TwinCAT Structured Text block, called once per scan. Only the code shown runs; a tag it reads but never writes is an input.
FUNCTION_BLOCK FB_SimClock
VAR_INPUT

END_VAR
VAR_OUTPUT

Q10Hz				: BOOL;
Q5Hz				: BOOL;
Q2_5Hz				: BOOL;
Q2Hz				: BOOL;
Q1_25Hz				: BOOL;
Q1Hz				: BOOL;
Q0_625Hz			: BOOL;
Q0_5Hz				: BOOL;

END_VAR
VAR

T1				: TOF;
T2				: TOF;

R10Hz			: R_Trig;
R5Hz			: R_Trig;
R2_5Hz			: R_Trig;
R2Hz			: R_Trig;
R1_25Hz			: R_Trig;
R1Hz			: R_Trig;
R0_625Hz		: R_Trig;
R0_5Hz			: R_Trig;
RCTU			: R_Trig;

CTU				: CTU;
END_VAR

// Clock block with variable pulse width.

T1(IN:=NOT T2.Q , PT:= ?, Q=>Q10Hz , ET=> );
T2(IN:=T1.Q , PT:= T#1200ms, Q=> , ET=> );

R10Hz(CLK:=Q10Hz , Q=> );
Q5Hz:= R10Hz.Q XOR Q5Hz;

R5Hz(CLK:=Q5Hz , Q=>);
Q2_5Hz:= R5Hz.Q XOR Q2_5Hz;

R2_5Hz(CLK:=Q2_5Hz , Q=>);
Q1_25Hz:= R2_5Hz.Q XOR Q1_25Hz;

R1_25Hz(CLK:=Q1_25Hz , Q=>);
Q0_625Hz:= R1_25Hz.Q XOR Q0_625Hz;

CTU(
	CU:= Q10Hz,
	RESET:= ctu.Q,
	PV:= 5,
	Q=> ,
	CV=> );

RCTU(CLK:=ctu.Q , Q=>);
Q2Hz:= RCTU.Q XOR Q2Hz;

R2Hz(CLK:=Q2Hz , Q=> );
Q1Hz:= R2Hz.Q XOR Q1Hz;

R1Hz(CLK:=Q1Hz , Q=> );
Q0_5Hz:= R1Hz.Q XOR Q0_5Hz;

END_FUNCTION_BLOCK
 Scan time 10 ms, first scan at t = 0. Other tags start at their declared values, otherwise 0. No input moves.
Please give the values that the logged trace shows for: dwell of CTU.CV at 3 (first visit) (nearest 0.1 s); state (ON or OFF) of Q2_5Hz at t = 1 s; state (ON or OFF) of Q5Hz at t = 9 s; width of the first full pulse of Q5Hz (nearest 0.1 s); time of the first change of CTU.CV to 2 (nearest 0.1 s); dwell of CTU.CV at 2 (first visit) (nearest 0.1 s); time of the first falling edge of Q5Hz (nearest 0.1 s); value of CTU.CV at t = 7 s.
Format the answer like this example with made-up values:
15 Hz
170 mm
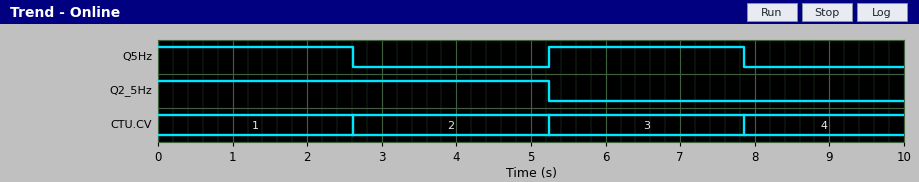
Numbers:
2.6 s
ON
OFF
2.6 s
2.6 s
2.6 s
2.6 s
3
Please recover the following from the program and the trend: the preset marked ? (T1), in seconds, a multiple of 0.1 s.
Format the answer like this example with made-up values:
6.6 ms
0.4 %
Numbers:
1.4 s
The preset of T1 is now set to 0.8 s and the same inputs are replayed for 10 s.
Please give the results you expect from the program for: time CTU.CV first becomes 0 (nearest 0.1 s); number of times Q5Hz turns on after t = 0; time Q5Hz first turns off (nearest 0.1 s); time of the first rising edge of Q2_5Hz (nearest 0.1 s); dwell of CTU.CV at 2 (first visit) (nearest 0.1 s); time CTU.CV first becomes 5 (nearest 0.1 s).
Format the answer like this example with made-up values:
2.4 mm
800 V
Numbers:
8.1 s
2
2.0 s
8.1 s
2.0 s
8.1 s
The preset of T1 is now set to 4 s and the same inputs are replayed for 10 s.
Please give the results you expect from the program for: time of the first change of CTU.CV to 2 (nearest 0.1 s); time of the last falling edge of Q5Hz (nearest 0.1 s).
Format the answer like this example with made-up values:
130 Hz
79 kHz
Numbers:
5.2 s
5.2 s
